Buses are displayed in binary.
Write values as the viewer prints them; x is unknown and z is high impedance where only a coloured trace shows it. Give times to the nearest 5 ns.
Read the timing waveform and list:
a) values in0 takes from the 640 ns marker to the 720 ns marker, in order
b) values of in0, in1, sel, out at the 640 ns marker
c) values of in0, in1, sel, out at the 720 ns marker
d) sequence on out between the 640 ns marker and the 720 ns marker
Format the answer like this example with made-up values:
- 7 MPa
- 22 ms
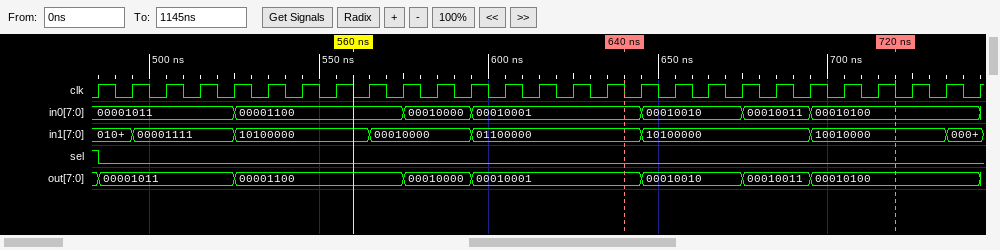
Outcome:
- 00010001, 00010010, 00010011, 00010100
- in0=00010001, in1=01100000, sel=0, out=00010001
- in0=00010100, in1=10010000, sel=0, out=00010100
- 00010001, 00010010, 00010011, 00010100
